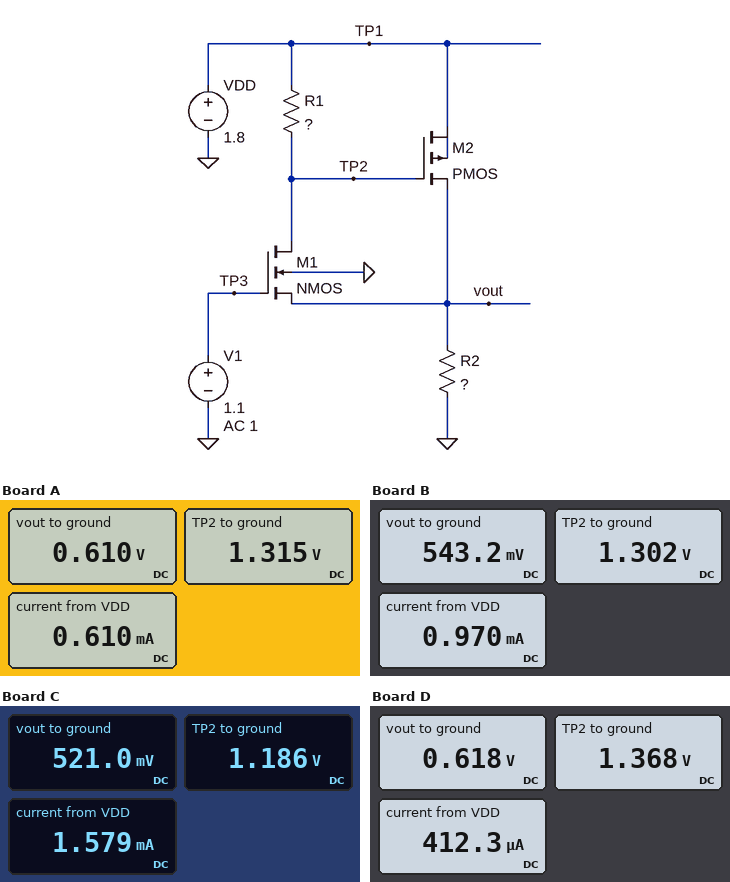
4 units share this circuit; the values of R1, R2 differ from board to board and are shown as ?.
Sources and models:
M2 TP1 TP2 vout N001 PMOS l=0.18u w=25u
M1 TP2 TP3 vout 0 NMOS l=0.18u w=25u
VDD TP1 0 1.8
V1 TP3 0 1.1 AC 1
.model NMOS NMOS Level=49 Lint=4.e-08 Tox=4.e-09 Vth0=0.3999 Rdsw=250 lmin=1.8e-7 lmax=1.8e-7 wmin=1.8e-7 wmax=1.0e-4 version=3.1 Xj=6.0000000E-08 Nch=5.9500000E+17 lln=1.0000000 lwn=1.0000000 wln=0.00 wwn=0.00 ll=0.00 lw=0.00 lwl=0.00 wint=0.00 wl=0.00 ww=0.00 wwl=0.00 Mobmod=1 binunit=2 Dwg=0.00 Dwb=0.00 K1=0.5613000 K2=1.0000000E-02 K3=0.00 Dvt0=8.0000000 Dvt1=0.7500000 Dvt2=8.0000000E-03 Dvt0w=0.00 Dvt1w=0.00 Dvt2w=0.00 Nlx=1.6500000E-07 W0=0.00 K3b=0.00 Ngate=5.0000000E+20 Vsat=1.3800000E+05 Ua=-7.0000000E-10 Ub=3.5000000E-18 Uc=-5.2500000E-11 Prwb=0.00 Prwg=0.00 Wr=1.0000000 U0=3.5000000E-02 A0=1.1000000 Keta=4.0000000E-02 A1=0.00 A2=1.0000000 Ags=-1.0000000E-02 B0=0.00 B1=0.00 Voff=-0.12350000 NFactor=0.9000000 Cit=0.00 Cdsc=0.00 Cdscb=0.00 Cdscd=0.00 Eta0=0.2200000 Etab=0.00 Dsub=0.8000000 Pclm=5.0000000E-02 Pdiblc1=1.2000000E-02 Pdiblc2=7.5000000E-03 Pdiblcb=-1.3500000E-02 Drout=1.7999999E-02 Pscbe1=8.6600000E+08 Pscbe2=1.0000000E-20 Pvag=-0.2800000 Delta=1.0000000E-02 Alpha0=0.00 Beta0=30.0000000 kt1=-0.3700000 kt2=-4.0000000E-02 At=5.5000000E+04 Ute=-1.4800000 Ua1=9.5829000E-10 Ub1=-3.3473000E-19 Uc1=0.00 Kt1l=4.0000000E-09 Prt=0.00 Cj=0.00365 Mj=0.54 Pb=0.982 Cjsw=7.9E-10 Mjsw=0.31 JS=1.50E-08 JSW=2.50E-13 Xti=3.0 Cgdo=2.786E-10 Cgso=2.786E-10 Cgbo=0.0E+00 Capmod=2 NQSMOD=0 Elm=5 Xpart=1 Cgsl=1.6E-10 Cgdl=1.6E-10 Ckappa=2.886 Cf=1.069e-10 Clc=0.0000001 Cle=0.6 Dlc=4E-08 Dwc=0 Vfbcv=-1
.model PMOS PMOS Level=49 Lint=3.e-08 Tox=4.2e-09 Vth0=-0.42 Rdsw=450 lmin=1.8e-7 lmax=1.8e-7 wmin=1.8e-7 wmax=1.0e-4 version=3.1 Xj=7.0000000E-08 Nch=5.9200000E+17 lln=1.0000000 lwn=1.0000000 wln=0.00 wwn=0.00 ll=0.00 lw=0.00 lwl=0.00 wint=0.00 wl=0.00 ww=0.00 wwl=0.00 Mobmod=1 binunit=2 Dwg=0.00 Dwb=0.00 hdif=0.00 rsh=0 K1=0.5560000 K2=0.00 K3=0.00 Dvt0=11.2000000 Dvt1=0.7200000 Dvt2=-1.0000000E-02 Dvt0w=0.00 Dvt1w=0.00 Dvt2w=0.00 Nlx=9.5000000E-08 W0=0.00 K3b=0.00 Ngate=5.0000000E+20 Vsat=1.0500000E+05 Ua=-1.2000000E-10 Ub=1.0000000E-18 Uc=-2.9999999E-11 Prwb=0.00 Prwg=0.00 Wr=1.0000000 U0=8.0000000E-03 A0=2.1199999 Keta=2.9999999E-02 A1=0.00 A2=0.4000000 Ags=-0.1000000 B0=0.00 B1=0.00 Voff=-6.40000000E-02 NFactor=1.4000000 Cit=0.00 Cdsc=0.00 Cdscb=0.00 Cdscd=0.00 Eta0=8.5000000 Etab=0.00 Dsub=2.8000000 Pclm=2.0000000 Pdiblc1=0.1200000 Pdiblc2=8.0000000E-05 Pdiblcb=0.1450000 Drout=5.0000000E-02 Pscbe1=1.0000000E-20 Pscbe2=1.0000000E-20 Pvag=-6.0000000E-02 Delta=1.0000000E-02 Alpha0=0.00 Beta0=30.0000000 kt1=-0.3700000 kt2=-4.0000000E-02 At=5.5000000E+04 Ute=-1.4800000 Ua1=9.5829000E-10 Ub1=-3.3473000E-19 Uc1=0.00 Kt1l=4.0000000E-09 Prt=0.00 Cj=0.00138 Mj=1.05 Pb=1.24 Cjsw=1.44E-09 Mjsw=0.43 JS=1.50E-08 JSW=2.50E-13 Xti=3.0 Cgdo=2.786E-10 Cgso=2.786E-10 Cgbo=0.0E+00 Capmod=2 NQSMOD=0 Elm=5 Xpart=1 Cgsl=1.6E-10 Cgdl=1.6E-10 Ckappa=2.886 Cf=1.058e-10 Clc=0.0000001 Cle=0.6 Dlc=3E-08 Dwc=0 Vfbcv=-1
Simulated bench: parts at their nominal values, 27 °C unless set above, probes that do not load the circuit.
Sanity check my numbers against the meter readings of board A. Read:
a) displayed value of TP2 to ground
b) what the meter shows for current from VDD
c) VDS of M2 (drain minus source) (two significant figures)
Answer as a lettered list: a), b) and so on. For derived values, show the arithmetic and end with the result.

a) 1.315 V
b) 0.610 mA
c) 1.8 V - 610 mV = 1.2 V
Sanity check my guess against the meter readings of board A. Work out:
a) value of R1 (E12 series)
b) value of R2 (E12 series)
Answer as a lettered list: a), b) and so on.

a) 3.9 kΩ
b) 1 kΩ
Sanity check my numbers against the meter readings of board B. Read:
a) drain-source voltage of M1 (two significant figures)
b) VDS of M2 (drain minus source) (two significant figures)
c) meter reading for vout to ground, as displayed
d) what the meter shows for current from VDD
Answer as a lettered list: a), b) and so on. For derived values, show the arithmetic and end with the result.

a) 1.302 V - 543.2 mV = 760 mV
b) 1.8 V - 543.2 mV = 1.3 V
c) 543.2 mV
d) 0.970 mA
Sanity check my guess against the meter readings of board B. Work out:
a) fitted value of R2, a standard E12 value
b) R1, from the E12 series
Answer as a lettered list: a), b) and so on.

a) 560 Ω
b) 1.2 kΩ
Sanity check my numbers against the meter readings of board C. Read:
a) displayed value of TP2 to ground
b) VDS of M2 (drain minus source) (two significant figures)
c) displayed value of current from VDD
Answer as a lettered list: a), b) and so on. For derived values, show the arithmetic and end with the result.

a) 1.186 V
b) 1.8 V - 521 mV = 1.3 V
c) 1.579 mA
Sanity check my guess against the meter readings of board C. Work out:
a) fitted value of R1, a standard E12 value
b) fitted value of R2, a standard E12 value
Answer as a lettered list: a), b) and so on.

a) 1.2 kΩ
b) 330 Ω
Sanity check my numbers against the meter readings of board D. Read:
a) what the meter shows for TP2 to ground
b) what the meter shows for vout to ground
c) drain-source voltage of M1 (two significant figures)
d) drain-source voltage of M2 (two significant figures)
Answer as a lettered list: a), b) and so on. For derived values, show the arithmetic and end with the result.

a) 1.368 V
b) 0.618 V
c) 1.368 V - 618 mV = 750 mV
d) 1.8 V - 618 mV = 1.2 V
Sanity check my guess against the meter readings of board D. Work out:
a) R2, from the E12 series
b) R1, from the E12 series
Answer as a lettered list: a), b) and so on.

a) 1.5 kΩ
b) 3.9 kΩ
